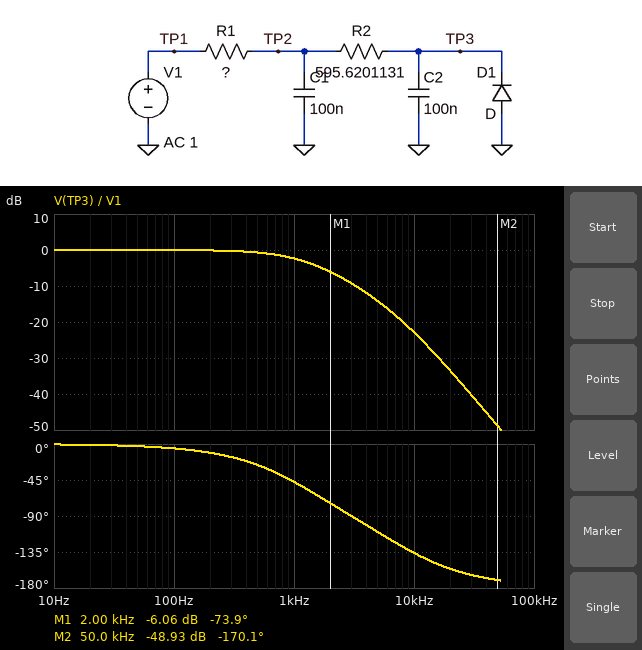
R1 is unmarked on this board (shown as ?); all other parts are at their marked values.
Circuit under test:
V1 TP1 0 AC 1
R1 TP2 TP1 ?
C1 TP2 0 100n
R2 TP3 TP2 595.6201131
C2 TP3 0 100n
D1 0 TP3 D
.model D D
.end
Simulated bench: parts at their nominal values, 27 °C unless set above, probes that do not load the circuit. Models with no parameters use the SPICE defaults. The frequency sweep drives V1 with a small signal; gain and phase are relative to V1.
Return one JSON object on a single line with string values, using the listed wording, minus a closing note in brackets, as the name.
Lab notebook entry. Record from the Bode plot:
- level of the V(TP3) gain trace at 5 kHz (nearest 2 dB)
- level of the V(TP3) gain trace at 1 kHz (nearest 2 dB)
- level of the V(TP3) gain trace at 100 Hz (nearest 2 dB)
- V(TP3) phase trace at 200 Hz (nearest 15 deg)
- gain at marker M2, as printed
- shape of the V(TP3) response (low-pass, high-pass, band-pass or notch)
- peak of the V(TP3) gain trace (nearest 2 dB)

{"level of the V(TP3) gain trace at 5 kHz": "-14 dB", "level of the V(TP3) gain trace at 1 kHz": "-2 dB", "level of the V(TP3) gain trace at 100 Hz": "0 dB", "V(TP3) phase trace at 200 Hz": "-15 deg", "gain at marker M2, as printed": "-48.93 dB", "shape of the V(TP3) response": "low-pass", "peak of the V(TP3) gain trace": "0 dB"}
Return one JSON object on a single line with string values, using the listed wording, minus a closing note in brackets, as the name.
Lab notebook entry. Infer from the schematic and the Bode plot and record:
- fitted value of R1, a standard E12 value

{"fitted value of R1, a standard E12 value": "470 Ω"}
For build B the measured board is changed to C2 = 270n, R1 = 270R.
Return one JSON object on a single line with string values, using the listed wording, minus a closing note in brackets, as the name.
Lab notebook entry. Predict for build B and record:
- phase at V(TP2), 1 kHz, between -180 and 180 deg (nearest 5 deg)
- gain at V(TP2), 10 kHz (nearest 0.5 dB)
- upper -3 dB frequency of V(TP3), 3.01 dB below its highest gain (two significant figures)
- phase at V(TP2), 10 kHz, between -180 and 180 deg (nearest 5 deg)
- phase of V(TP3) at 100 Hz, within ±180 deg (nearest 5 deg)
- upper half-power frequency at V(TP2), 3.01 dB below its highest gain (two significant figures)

{"phase at V(TP2), 1 kHz, between -180 and 180 deg": "-20 deg", "gain at V(TP2), 10 kHz": "-7.0 dB", "upper -3 dB frequency of V(TP3), 3.01 dB below its highest gain": "650 Hz", "phase at V(TP2), 10 kHz, between -180 and 180 deg": "-50 deg", "phase of V(TP3) at 100 Hz, within ±180 deg": "-10 deg", "upper half-power frequency at V(TP2), 3.01 dB below its highest gain": "1.6 kHz"}
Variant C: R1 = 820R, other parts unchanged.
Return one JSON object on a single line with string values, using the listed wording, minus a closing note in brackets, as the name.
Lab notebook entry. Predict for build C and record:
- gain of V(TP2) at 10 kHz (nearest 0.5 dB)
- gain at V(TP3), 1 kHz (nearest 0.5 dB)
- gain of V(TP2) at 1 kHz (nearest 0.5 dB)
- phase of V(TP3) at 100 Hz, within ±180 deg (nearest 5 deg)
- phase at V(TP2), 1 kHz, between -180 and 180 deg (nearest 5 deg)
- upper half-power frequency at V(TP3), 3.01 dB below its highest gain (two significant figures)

{"gain of V(TP2) at 10 kHz": "-15.5 dB", "gain at V(TP3), 1 kHz": "-4.0 dB", "gain of V(TP2) at 1 kHz": "-3.5 dB", "phase of V(TP3) at 100 Hz, within ±180 deg": "-10 deg", "phase at V(TP2), 1 kHz, between -180 and 180 deg": "-40 deg", "upper half-power frequency at V(TP3), 3.01 dB below its highest gain": "790 Hz"}
